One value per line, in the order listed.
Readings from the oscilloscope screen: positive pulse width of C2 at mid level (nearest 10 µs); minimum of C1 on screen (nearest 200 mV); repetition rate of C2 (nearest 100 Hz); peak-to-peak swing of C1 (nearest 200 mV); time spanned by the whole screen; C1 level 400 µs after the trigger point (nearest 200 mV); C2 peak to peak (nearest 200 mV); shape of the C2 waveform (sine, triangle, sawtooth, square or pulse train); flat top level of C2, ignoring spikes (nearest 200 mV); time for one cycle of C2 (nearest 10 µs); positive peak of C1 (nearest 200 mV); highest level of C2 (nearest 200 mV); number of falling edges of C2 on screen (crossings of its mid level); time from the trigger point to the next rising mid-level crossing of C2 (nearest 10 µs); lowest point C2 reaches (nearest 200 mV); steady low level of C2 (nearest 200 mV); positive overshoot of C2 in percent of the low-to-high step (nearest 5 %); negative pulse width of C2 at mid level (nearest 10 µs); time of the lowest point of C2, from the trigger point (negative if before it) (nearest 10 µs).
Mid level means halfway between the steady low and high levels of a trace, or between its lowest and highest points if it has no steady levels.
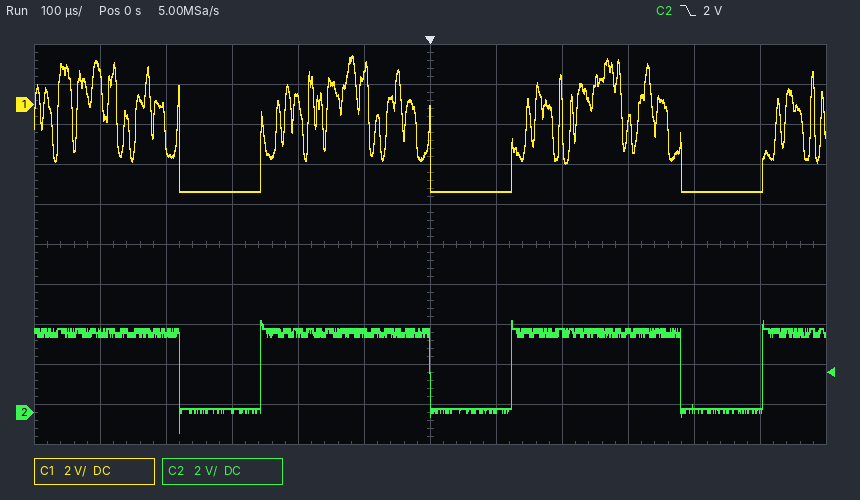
260 µs
-4.4 V
2.6 kHz
6.8 V
1.2 ms
-4.4 V
5.6 V
pulse train
4.0 V
380 µs
2.4 V
4.6 V
3
120 µs
-1.0 V
200 mV
15 %
120 µs
-380 µs
